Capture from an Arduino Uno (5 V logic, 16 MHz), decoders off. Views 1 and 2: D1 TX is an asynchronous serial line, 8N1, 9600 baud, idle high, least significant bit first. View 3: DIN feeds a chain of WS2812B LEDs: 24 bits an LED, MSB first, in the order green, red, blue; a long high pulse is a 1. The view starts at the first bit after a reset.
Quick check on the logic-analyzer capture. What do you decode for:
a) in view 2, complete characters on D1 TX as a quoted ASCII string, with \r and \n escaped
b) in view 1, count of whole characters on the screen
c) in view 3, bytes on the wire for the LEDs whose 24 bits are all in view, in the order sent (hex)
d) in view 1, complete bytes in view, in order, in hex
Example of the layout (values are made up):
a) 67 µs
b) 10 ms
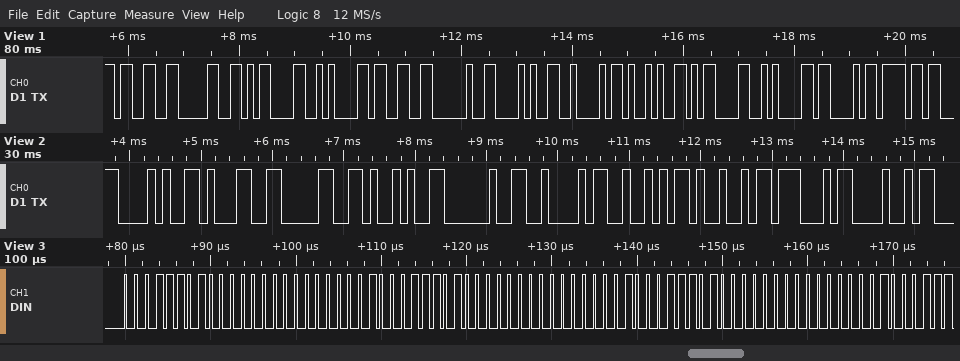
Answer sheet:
a) "(10) BRIGH"
b) 13
c) 1D 00 01 1D 00 01 1D 00 01
d) 33 30 0D 0A 33 20 28 42 29 0D 0A 43 6F
